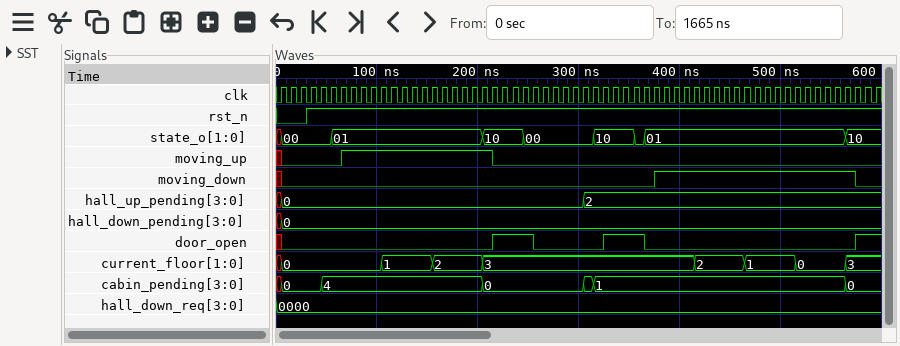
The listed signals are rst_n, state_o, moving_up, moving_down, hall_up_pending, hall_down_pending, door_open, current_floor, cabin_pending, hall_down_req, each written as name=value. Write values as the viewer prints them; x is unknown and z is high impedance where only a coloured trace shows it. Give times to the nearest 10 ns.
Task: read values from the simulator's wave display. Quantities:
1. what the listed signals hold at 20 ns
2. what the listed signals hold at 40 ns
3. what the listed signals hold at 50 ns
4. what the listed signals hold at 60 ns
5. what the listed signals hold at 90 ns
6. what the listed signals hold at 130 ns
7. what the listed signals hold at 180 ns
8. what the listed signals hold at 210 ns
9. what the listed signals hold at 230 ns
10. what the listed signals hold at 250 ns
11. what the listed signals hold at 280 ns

rst_n=0, state_o=00, moving_up=0, moving_down=0, hall_up_pending=0, hall_down_pending=0, door_open=0, current_floor=0, cabin_pending=0, hall_down_req=0000
rst_n=1, state_o=00, moving_up=0, moving_down=0, hall_up_pending=0, hall_down_pending=0, door_open=0, current_floor=0, cabin_pending=0, hall_down_req=0000
rst_n=1, state_o=00, moving_up=0, moving_down=0, hall_up_pending=0, hall_down_pending=0, door_open=0, current_floor=0, cabin_pending=4, hall_down_req=0000
rst_n=1, state_o=01, moving_up=0, moving_down=0, hall_up_pending=0, hall_down_pending=0, door_open=0, current_floor=0, cabin_pending=4, hall_down_req=0000
rst_n=1, state_o=01, moving_up=1, moving_down=0, hall_up_pending=0, hall_down_pending=0, door_open=0, current_floor=0, cabin_pending=4, hall_down_req=0000
rst_n=1, state_o=01, moving_up=1, moving_down=0, hall_up_pending=0, hall_down_pending=0, door_open=0, current_floor=1, cabin_pending=4, hall_down_req=0000
rst_n=1, state_o=01, moving_up=1, moving_down=0, hall_up_pending=0, hall_down_pending=0, door_open=0, current_floor=2, cabin_pending=4, hall_down_req=0000
rst_n=1, state_o=10, moving_up=1, moving_down=0, hall_up_pending=0, hall_down_pending=0, door_open=0, current_floor=3, cabin_pending=0, hall_down_req=0000
rst_n=1, state_o=10, moving_up=0, moving_down=0, hall_up_pending=0, hall_down_pending=0, door_open=1, current_floor=3, cabin_pending=0, hall_down_req=0000
rst_n=1, state_o=00, moving_up=0, moving_down=0, hall_up_pending=0, hall_down_pending=0, door_open=1, current_floor=3, cabin_pending=0, hall_down_req=0000
rst_n=1, state_o=00, moving_up=0, moving_down=0, hall_up_pending=0, hall_down_pending=0, door_open=0, current_floor=3, cabin_pending=0, hall_down_req=0000
